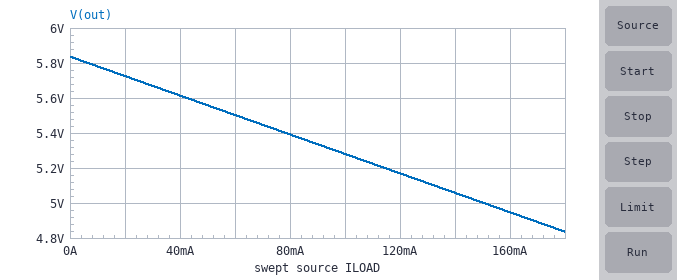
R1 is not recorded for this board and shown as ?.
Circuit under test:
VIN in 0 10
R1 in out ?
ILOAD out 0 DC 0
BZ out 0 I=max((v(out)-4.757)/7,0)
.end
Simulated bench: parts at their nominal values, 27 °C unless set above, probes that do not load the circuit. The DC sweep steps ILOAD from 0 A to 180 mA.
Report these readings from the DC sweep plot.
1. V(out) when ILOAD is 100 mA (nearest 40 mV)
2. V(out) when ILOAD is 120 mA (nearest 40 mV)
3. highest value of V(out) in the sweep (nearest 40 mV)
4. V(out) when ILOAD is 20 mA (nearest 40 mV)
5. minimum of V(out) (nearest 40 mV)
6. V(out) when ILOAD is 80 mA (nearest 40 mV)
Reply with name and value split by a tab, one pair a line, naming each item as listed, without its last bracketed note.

V(out) when ILOAD is 100 mA	5.28 V
V(out) when ILOAD is 120 mA	5.16 V
highest value of V(out) in the sweep	5.84 V
V(out) when ILOAD is 20 mA	5.72 V
minimum of V(out)	4.84 V
V(out) when ILOAD is 80 mA	5.40 V
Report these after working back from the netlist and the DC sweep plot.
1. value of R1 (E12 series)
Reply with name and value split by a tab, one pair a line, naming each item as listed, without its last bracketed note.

value of R1	27 Ω
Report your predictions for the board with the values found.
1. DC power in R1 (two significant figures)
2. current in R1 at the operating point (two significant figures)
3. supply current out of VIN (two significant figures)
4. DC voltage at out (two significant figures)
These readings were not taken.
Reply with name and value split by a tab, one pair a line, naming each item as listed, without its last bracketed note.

DC power in R1	640 mW
current in R1 at the operating point	150 mA
supply current out of VIN	150 mA
DC voltage at out	5.8 V
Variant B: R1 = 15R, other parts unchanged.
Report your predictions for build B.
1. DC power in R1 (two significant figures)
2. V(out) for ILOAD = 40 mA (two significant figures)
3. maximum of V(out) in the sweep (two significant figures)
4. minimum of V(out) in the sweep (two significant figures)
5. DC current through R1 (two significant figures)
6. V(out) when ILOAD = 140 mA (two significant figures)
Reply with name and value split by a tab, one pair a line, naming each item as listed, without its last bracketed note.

DC power in R1	850 mW
V(out) for ILOAD = 40 mA	6.2 V
maximum of V(out) in the sweep	6.4 V
minimum of V(out) in the sweep	5.6 V
DC current through R1	240 mA
V(out) when ILOAD = 140 mA	5.8 V
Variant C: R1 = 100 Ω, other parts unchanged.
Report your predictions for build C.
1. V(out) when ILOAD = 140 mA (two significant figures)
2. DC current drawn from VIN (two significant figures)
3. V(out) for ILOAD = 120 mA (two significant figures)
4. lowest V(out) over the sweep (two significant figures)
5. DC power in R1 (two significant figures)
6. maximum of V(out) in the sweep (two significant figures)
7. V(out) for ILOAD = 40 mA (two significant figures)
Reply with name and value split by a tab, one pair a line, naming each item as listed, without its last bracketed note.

V(out) when ILOAD = 140 mA	-4.0 V
DC current drawn from VIN	49 mA
V(out) for ILOAD = 120 mA	-2.0 V
lowest V(out) over the sweep	-8.0 V
DC power in R1	240 mW
maximum of V(out) in the sweep	5.1 V
V(out) for ILOAD = 40 mA	4.8 V
